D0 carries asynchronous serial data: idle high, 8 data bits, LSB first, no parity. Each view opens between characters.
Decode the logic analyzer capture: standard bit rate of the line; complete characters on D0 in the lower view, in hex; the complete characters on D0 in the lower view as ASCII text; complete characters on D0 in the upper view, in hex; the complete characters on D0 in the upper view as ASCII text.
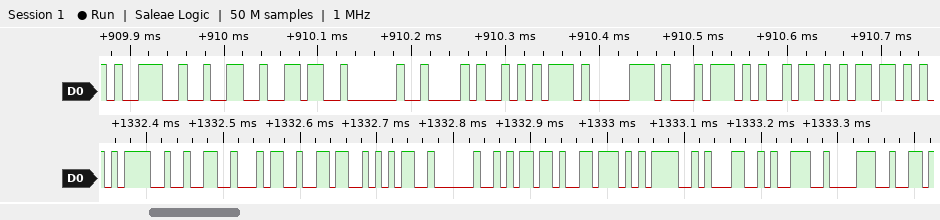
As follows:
115200 baud
3D, 32, 34, 36, 35, 20, 6D, 76, 3D, 31, 39, 38
"=2465 mv=198"
39, 32, 36, 20, 28, 75, 70, 74, 69, 6D
"926 (uptim"
